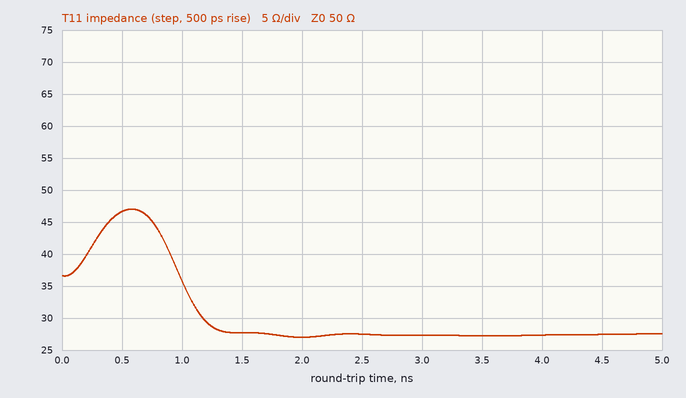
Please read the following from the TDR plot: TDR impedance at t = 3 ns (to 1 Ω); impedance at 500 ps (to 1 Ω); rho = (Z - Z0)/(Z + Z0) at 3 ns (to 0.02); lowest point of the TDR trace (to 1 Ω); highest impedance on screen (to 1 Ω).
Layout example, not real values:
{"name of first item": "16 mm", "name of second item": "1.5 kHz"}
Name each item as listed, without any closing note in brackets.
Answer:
{"TDR impedance at t = 3 ns": "27 Ω", "impedance at 500 ps": "47 Ω", "rho = (Z - Z0)/(Z + Z0) at 3 ns": "-0.30", "lowest point of the TDR trace": "27 Ω", "highest impedance on screen": "47 Ω"}
